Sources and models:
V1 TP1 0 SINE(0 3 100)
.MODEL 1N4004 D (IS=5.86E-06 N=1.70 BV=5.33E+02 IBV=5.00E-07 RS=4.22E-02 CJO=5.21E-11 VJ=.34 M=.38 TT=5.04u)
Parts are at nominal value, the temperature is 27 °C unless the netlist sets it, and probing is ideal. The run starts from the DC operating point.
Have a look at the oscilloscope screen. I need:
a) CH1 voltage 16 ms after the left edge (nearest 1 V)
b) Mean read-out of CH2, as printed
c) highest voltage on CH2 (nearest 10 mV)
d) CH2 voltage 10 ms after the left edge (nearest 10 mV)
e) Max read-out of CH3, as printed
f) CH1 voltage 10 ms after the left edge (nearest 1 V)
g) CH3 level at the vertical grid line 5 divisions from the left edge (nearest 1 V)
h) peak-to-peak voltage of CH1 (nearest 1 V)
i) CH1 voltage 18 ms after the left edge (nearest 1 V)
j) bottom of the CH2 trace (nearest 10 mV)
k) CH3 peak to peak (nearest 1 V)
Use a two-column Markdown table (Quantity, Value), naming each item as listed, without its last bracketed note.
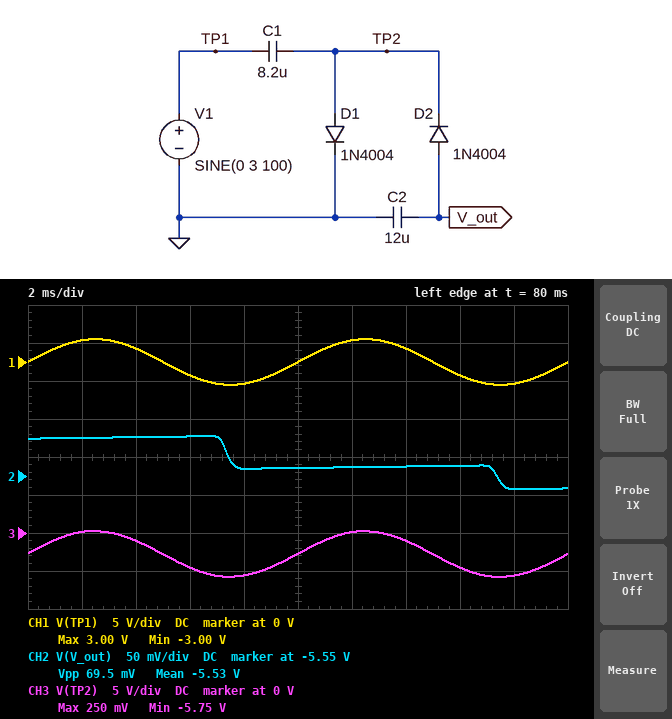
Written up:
| Quantity | Value |
|---|---|
| CH1 voltage 16 ms after the left edge | -2 V |
| Mean read-out of CH2, as printed | -5.53 V |
| highest voltage on CH2 | -5.50 V |
| CH2 voltage 10 ms after the left edge | -5.54 V |
| Max read-out of CH3, as printed | 250 mV |
| CH1 voltage 10 ms after the left edge | 0 V |
| CH3 level at the vertical grid line 5 divisions from the left edge | -3 V |
| peak-to-peak voltage of CH1 | 6 V |
| CH1 voltage 18 ms after the left edge | -3 V |
| bottom of the CH2 trace | -5.57 V |
| CH3 peak to peak | 6 V |
